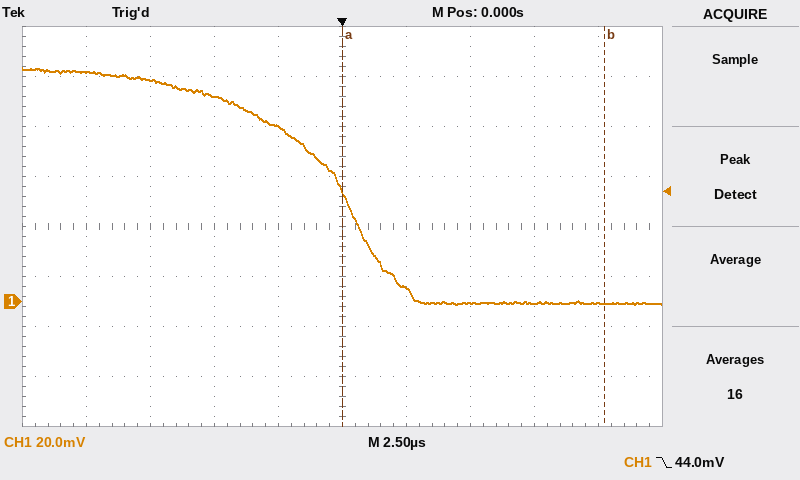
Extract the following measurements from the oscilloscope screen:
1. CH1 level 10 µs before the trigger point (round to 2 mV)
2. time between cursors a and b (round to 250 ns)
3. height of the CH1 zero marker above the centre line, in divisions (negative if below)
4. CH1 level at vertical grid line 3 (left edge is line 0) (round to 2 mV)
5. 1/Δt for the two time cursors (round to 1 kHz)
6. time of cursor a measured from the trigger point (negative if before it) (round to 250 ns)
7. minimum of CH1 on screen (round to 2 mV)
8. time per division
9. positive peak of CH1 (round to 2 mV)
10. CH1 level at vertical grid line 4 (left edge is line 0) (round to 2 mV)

92 mV
10.25 µs
-1.5 div
82 mV
98 kHz
0.00 µs
-2 mV
2.5 µs
94 mV
70 mV
